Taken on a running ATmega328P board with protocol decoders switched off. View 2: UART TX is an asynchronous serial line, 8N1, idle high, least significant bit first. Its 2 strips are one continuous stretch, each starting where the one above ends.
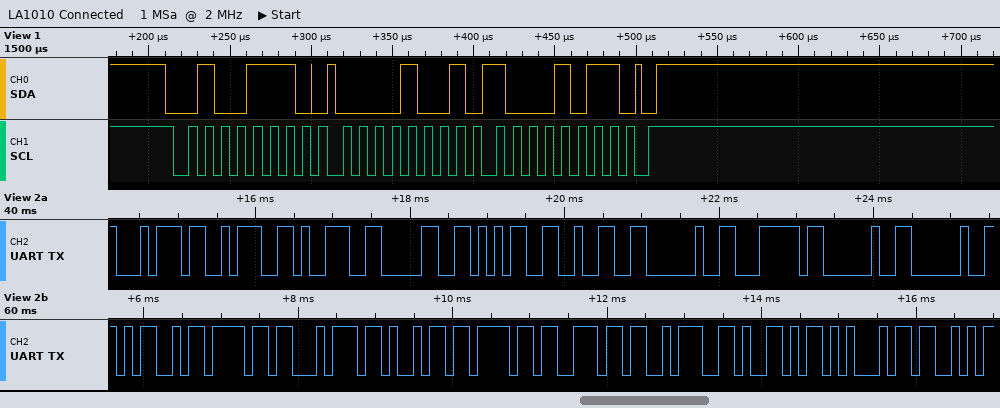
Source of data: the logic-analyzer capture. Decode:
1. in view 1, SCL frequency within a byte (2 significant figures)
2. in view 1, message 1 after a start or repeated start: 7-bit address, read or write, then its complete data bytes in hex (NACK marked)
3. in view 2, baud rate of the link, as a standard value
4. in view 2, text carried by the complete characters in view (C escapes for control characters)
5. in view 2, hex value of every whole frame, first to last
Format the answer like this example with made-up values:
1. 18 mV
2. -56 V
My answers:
1. 100 kHz
2. 0x27 write: 09 8B
3. 9600 baud
4. "t:9052 |  Motion:YES"
5. 74 3A 39 30 35 32 20 7C 20 20 4D 6F 74 69 6F 6E 3A 59 45 53
